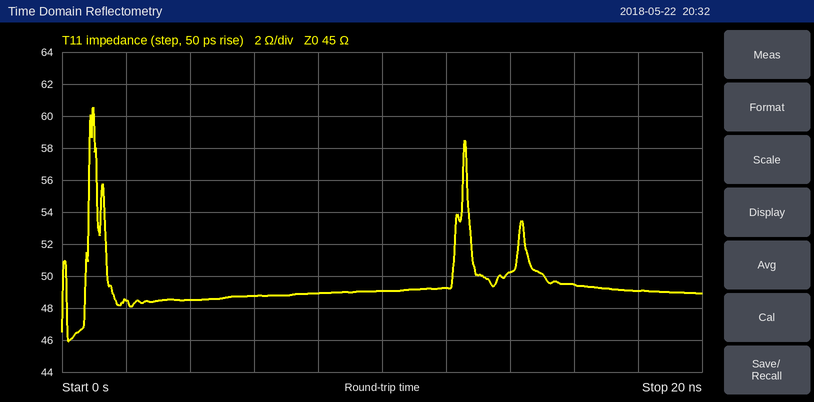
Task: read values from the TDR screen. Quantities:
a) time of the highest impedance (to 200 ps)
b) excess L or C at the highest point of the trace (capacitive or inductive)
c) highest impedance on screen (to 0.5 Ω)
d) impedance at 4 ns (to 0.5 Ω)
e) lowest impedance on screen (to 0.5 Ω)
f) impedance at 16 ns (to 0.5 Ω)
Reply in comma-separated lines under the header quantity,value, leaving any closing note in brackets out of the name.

quantity,value
time of the highest impedance,1.0 ns
excess L or C at the highest point of the trace,inductive
highest impedance on screen,60.5 Ω
impedance at 4 ns,48.5 Ω
lowest impedance on screen,46.0 Ω
impedance at 16 ns,49.5 Ω
